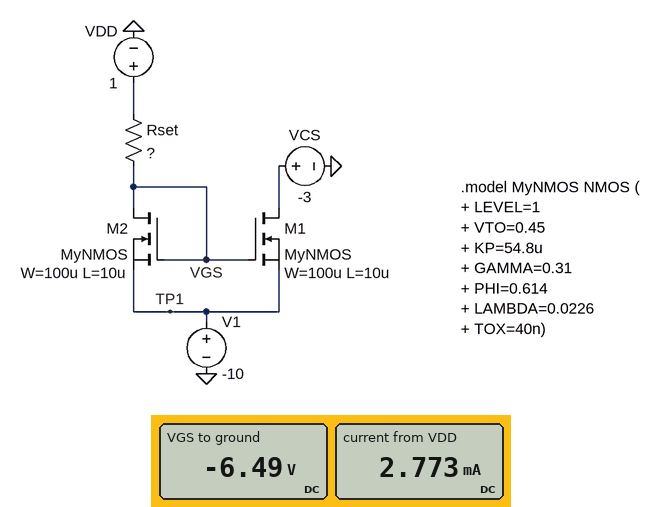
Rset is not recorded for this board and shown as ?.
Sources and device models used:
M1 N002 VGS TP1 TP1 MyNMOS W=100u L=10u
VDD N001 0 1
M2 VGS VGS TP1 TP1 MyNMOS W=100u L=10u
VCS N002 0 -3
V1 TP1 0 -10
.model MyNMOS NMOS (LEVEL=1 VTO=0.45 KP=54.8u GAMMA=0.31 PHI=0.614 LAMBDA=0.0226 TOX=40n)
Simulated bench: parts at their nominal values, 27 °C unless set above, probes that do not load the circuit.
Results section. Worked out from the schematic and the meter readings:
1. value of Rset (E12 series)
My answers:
2.7 kΩ
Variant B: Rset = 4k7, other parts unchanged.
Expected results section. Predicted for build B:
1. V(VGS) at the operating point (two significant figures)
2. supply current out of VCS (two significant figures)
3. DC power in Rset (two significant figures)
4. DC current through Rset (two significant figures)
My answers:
-7.1 V
1.9 mA
14 mW
1.7 mA
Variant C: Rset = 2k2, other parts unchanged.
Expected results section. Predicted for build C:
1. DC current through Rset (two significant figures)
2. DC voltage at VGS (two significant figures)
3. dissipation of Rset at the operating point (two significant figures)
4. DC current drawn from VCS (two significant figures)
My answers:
3.3 mA
-6.2 V
24 mW
3.5 mA
